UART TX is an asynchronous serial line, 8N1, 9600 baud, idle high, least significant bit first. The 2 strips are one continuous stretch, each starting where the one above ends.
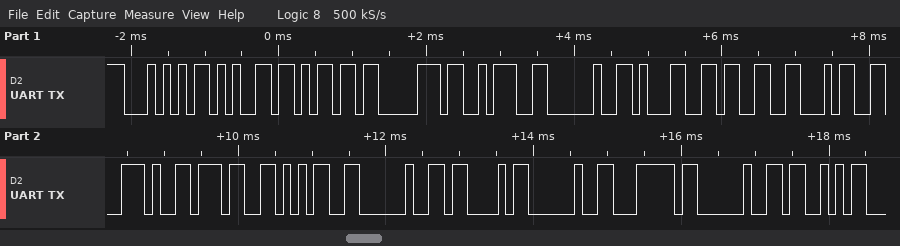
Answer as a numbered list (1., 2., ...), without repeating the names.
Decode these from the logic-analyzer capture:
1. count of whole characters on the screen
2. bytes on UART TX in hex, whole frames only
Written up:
1. 18
2. 0x54 0x65 0x6D 0x70 0x3A 0x20 0x31 0x33 0x34 0x2E 0x37 0x35 0x20 0x43 0x20 0x7C 0x20 0x53
